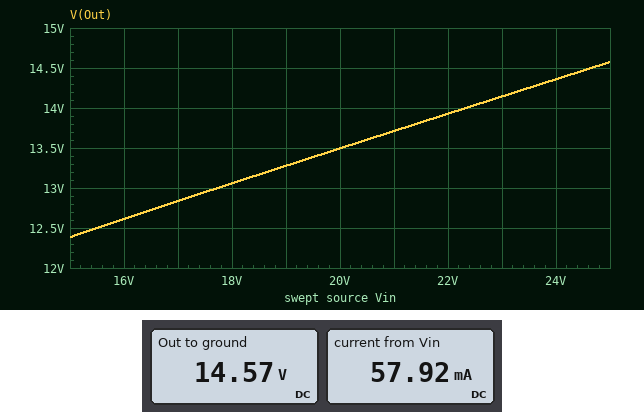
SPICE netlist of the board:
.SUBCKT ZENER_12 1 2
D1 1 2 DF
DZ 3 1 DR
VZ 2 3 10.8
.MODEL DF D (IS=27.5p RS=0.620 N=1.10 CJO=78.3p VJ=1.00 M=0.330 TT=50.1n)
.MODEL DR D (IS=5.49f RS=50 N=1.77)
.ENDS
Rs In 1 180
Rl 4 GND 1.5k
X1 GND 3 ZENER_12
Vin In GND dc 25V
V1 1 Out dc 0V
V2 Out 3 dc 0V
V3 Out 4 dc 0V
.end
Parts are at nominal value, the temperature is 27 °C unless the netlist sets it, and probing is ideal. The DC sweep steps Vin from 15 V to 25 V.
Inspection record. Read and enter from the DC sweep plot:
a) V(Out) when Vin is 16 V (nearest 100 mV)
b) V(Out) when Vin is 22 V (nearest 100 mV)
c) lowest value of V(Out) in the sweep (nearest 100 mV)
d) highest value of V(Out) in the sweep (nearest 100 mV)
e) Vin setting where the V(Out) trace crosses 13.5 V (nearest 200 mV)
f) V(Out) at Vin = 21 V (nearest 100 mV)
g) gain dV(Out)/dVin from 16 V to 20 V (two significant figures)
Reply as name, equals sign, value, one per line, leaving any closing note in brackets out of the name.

V(Out) when Vin is 16 V = 12.6 V
V(Out) when Vin is 22 V = 13.9 V
lowest value of V(Out) in the sweep = 12.4 V
highest value of V(Out) in the sweep = 14.6 V
Vin setting where the V(Out) trace crosses 13.5 V = 20.0 V
V(Out) at Vin = 21 V = 13.7 V
gain dV(Out)/dVin from 16 V to 20 V = 0.22 V/V
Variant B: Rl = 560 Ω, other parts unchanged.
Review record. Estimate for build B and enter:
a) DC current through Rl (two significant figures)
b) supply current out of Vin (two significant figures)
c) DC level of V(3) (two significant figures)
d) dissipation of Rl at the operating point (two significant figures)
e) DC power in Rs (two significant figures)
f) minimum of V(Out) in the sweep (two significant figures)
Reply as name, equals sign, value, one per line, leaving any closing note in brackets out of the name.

DC current through Rl = 25 mA
supply current out of Vin = 61 mA
DC level of V(3) = 14 V
dissipation of Rl at the operating point = 350 mW
DC power in Rs = 680 mW
minimum of V(Out) in the sweep = 11 V
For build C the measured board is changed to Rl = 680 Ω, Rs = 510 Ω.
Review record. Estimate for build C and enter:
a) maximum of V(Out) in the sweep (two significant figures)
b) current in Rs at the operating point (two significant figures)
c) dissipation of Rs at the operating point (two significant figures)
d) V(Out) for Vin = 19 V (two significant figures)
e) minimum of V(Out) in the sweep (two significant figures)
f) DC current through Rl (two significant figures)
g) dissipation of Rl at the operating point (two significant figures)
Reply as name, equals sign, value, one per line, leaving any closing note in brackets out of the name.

maximum of V(Out) in the sweep = 12 V
current in Rs at the operating point = 25 mA
dissipation of Rs at the operating point = 310 mW
V(Out) for Vin = 19 V = 11 V
minimum of V(Out) in the sweep = 8.6 V
DC current through Rl = 18 mA
dissipation of Rl at the operating point = 230 mW
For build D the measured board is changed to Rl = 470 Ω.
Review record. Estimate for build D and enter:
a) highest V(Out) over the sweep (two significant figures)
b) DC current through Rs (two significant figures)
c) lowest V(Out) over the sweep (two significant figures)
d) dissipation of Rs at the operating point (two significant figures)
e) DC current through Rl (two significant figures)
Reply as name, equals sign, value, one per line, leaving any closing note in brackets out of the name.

highest V(Out) over the sweep = 14 V
DC current through Rs = 62 mA
lowest V(Out) over the sweep = 11 V
dissipation of Rs at the operating point = 700 mW
DC current through Rl = 29 mA
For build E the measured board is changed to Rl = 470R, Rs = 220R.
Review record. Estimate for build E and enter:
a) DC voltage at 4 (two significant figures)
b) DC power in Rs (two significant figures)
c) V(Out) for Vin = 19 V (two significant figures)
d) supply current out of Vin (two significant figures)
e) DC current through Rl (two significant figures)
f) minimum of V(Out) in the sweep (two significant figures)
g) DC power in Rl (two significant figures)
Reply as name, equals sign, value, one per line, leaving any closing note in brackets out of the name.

DC voltage at 4 = 13 V
DC power in Rs = 620 mW
V(Out) for Vin = 19 V = 12 V
supply current out of Vin = 53 mA
DC current through Rl = 28 mA
minimum of V(Out) in the sweep = 10 V
DC power in Rl = 380 mW
